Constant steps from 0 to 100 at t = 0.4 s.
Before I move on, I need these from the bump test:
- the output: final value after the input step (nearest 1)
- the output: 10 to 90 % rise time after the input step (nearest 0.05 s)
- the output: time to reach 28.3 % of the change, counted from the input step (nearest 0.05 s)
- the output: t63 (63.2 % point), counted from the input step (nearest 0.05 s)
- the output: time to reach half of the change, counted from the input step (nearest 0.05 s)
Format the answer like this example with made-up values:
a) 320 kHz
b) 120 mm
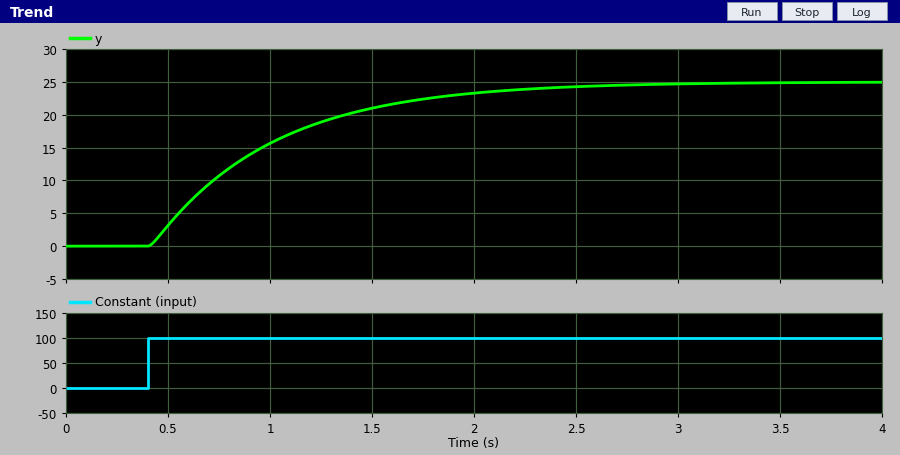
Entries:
a) 25
b) 1.30 s
c) 0.20 s
d) 0.60 s
e) 0.45 s
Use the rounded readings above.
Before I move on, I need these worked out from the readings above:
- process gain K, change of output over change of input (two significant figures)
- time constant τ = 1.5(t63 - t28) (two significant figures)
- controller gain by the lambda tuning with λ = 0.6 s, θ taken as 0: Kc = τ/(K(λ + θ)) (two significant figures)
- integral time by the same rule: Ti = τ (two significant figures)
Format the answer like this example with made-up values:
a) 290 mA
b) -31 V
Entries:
a) 0.25
b) 0.60 s
c) 4.0
d) 0.60 s
